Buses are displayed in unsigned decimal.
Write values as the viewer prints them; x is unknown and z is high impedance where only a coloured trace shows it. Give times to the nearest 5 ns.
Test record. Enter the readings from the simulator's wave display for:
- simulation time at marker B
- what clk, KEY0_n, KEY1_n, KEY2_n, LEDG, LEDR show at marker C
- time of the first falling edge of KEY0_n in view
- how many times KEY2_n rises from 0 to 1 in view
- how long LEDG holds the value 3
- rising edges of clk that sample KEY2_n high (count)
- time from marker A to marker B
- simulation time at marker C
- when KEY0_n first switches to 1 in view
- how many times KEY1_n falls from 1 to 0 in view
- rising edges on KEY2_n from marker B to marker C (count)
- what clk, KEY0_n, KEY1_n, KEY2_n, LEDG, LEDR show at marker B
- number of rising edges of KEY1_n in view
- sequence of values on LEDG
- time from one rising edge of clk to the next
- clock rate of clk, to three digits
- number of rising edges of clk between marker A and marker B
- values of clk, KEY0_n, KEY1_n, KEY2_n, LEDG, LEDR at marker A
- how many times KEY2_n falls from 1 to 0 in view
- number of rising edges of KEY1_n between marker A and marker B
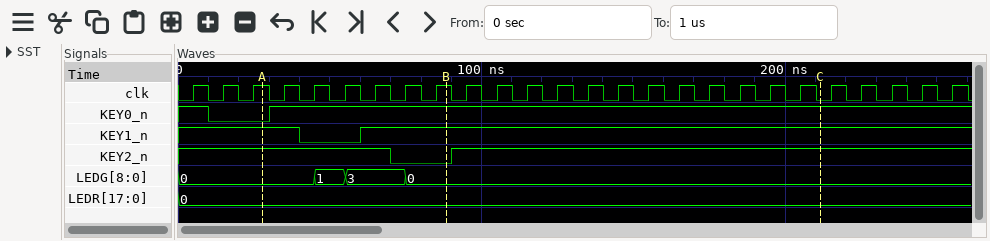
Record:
90 ns
clk=0, KEY0_n=1, KEY1_n=1, KEY2_n=1, LEDG=0, LEDR=0
10 ns
1
20 ns
24
60 ns
210 ns
30 ns
1
1
clk=1, KEY0_n=1, KEY1_n=1, KEY2_n=0, LEDG=0, LEDR=0
1
0, 1, 3, 0
10 ns
100 MHz
6
clk=1, KEY0_n=0, KEY1_n=1, KEY2_n=1, LEDG=0, LEDR=0
1
1
